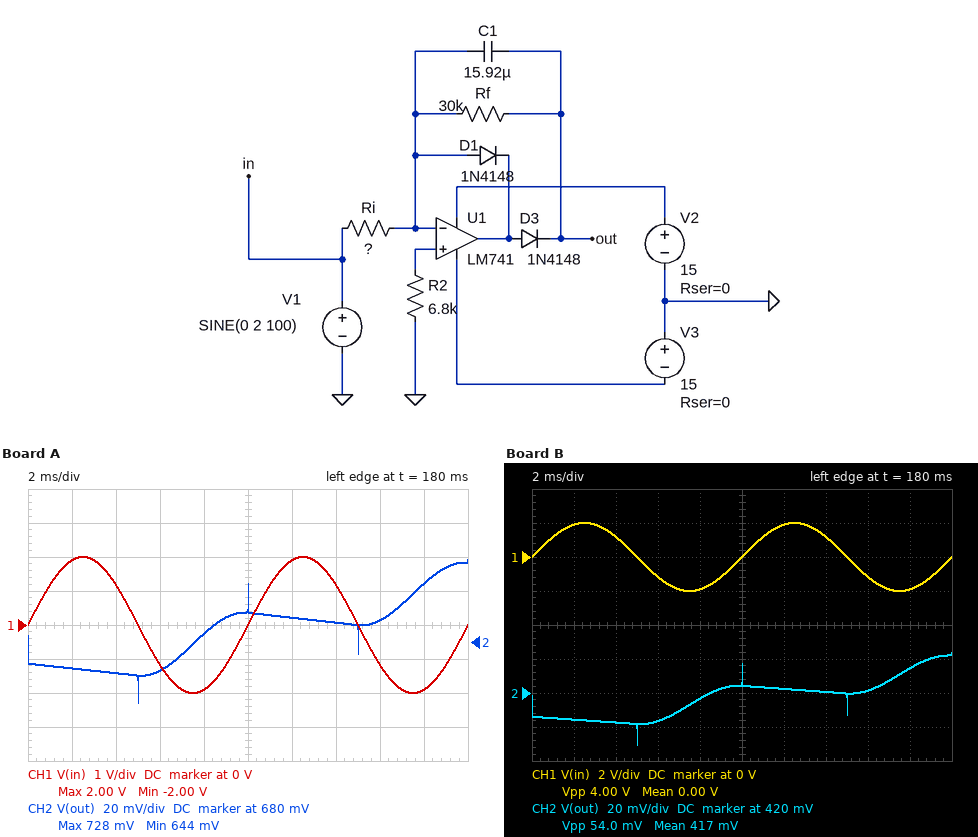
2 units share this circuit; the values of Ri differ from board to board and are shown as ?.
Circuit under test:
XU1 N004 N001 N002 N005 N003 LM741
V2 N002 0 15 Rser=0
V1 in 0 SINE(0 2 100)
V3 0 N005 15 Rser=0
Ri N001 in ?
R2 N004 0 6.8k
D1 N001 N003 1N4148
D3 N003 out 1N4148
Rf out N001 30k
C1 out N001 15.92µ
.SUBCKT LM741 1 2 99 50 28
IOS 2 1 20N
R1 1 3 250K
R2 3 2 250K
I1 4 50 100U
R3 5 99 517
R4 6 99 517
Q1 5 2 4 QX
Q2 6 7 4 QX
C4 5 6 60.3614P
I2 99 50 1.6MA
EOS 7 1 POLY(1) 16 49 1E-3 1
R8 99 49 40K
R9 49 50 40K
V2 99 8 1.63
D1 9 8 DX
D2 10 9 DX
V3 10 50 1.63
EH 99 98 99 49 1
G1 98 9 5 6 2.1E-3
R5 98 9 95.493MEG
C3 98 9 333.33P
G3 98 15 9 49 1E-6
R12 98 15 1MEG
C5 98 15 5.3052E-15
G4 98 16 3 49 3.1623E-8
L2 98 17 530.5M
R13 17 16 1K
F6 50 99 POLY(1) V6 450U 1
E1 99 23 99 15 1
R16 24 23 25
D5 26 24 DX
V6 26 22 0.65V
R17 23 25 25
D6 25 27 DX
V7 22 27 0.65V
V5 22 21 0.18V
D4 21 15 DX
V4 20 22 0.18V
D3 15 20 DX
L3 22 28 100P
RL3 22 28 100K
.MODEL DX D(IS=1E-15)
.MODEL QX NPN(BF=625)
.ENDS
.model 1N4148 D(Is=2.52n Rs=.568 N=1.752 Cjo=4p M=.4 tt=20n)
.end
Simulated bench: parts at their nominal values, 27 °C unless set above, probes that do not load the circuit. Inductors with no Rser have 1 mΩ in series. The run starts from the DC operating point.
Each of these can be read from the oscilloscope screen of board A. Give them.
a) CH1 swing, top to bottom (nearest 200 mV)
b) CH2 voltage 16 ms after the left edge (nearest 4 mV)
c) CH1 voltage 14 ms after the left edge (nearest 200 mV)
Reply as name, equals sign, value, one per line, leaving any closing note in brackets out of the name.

CH1 swing, top to bottom = 4.0 V
CH2 voltage 16 ms after the left edge = 692 mV
CH1 voltage 14 ms after the left edge = 1.2 V
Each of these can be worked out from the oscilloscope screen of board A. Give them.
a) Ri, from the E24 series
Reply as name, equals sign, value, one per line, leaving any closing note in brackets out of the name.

Ri, from the E24 series = 9.1 kΩ
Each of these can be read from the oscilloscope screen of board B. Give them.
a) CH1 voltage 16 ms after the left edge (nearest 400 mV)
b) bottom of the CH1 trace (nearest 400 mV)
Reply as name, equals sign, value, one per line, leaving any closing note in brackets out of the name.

CH1 voltage 16 ms after the left edge = -1.2 V
bottom of the CH1 trace = -2.0 V
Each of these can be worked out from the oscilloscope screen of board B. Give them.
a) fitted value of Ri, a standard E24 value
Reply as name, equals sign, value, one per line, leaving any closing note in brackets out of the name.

fitted value of Ri, a standard E24 value = 15 kΩ
